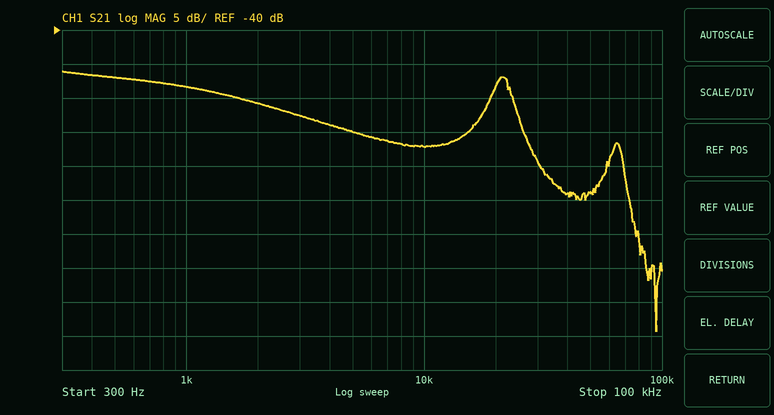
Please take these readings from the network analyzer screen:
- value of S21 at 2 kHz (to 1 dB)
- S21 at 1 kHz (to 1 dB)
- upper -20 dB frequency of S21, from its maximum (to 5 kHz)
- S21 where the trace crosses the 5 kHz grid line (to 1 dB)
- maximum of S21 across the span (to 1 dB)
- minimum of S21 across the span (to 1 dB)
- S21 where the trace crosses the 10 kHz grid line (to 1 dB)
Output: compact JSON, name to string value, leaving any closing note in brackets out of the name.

{"value of S21 at 2 kHz": "-51 dB", "S21 at 1 kHz": "-48 dB", "upper -20 dB frequency of S21, from its maximum": "75 kHz", "S21 where the trace crosses the 5 kHz grid line": "-55 dB", "maximum of S21 across the span": "-46 dB", "minimum of S21 across the span": "-84 dB", "S21 where the trace crosses the 10 kHz grid line": "-57 dB"}
